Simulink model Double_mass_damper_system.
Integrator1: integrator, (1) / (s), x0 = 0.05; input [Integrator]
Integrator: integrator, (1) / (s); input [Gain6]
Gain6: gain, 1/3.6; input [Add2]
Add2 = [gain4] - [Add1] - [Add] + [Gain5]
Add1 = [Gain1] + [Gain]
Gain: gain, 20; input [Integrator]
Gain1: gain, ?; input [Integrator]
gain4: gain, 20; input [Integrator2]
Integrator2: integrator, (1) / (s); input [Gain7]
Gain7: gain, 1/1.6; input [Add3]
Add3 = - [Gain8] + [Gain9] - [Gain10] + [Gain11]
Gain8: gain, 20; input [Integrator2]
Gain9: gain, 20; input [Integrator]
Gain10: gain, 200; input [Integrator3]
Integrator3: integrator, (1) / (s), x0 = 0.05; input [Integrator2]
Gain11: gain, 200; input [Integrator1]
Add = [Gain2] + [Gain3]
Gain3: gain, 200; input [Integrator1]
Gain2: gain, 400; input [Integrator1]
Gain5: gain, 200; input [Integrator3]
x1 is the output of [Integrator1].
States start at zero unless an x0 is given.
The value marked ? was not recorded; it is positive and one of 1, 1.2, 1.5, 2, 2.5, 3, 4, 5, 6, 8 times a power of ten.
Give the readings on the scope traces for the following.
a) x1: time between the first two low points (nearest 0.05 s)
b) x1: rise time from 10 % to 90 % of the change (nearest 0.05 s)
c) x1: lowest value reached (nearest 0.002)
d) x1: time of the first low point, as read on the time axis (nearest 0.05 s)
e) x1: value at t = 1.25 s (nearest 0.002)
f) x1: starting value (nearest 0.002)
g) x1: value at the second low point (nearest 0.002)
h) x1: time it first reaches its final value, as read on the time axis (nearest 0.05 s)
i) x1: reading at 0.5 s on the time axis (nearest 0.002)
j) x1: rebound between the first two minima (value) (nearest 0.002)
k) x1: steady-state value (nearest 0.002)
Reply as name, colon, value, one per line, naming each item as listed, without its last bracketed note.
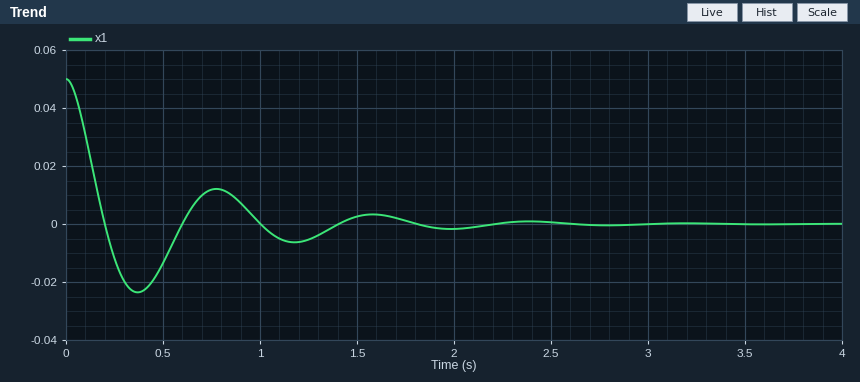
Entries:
x1: time between the first two low points: 0.80 s
x1: rise time from 10 % to 90 % of the change: 0.15 s
x1: lowest value reached: -0.024
x1: time of the first low point, as read on the time axis: 0.35 s
x1: value at t = 1.25 s: -0.006
x1: starting value: 0.050
x1: value at the second low point: -0.006
x1: time it first reaches its final value, as read on the time axis: 0.20 s
x1: reading at 0.5 s on the time axis: -0.014
x1: rebound between the first two minima (value): 0.012
x1: steady-state value: 0.000
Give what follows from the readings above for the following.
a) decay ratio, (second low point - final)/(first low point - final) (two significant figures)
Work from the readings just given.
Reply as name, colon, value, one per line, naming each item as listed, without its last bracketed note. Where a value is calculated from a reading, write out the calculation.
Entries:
decay ratio, (second low point - final)/(first low point - final): (-0.006 - 0) / (-0.024 - 0) = 0.25
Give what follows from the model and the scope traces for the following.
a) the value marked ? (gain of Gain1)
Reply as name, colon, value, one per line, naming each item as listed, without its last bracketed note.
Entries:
the value marked ?: 15
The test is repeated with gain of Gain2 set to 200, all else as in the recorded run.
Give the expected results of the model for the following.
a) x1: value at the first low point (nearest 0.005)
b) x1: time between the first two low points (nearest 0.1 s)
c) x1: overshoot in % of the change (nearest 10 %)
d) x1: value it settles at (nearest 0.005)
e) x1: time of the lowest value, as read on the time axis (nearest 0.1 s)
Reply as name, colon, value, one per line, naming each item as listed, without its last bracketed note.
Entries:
x1: value at the first low point: -0.020
x1: time between the first two low points: 1.1 s
x1: overshoot in % of the change: 40 %
x1: value it settles at: 0.000
x1: time of the lowest value, as read on the time axis: 0.5 s
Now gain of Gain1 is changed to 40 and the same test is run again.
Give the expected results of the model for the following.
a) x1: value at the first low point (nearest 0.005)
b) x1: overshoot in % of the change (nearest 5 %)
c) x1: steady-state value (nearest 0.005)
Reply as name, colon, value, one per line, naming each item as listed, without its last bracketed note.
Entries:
x1: value at the first low point: -0.010
x1: overshoot in % of the change: 20 %
x1: steady-state value: 0.000
